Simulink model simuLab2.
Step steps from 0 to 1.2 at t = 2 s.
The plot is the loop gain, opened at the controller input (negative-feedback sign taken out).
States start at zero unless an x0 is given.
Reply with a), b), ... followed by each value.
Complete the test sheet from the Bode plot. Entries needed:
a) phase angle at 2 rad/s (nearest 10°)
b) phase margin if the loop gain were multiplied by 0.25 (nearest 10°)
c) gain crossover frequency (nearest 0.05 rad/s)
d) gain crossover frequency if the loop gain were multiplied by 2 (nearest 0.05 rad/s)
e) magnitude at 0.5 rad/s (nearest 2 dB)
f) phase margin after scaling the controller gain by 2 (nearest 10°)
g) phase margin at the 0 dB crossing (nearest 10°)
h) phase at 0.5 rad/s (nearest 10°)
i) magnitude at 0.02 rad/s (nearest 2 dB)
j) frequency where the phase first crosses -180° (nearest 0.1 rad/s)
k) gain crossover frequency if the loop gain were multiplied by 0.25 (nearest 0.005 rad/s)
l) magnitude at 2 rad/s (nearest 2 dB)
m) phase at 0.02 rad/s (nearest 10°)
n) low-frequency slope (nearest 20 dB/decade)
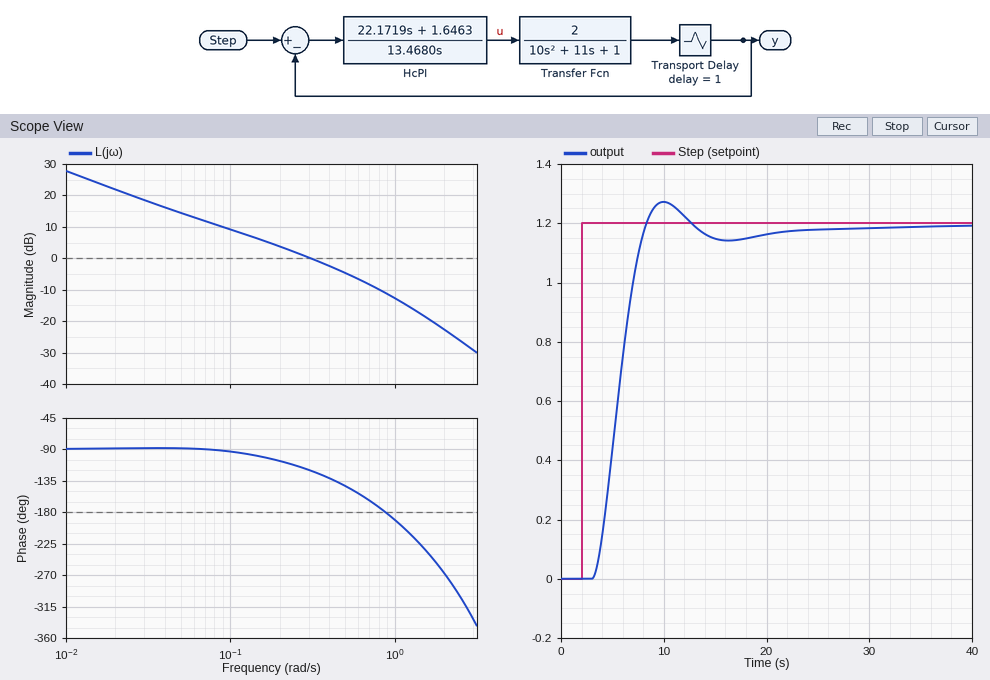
a) -270°
b) 90°
c) 0.30 rad/s
d) 0.55 rad/s
e) -4 dB
f) 30°
g) 60°
h) -140°
i) 22 dB
j) 0.9 rad/s
k) 0.070 rad/s
l) -22 dB
m) -90°
n) -20 dB/decade
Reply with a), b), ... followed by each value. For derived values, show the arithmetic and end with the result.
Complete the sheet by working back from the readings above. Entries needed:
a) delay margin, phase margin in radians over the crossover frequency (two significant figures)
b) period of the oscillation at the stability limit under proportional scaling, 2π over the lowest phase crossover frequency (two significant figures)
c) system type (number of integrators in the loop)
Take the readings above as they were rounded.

a) 60 × π / 180 / 0.3 = 3.5 s
b) 2π / 0.9 = 7.0 s
c) 1
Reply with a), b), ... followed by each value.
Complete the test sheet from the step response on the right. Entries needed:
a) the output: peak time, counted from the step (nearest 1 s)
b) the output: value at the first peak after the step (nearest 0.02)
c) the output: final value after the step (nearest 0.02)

a) 8 s
b) 1.28
c) 1.20
